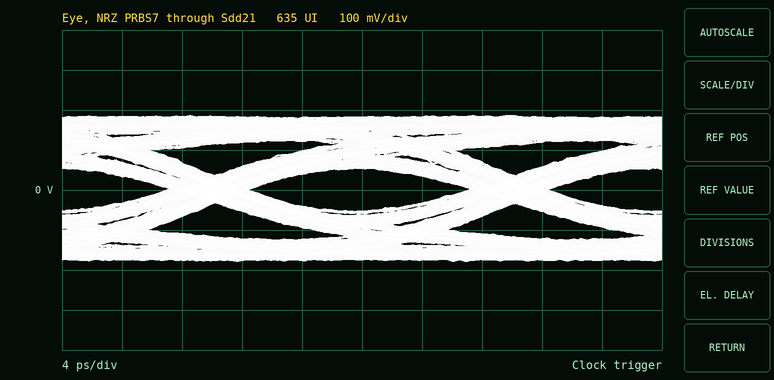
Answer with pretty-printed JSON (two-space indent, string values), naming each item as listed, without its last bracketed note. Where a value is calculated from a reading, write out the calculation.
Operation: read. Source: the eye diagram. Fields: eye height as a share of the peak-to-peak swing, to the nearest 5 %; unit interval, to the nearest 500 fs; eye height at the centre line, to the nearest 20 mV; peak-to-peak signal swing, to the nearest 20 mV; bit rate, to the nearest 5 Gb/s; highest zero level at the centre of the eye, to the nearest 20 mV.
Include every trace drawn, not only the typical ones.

{
  "eye height as a share of the peak-to-peak swing, to the nearest 5 %": "100 mV / 360 mV ≈ 27.8 %, so 30 % to the nearest 5 %",
  "unit interval, to the nearest 500 fs": "20.0 ps",
  "eye height at the centre line, to the nearest 20 mV": "100 mV",
  "peak-to-peak signal swing, to the nearest 20 mV": "360 mV",
  "bit rate, to the nearest 5 Gb/s": "50 Gb/s",
  "highest zero level at the centre of the eye, to the nearest 20 mV": "-60 mV"
}
